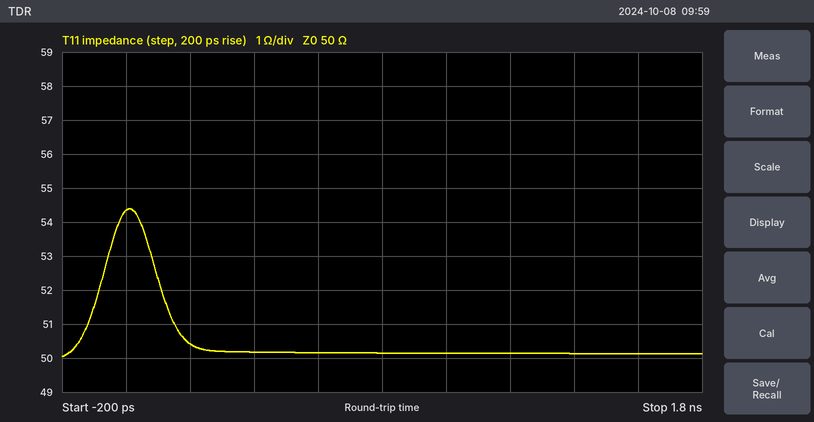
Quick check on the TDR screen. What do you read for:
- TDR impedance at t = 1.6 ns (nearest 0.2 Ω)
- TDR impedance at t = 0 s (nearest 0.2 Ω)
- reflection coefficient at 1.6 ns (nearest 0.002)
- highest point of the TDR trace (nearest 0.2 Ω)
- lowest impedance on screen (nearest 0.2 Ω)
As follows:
50.2 Ω
54.4 Ω
+0.002
54.4 Ω
50.0 Ω
